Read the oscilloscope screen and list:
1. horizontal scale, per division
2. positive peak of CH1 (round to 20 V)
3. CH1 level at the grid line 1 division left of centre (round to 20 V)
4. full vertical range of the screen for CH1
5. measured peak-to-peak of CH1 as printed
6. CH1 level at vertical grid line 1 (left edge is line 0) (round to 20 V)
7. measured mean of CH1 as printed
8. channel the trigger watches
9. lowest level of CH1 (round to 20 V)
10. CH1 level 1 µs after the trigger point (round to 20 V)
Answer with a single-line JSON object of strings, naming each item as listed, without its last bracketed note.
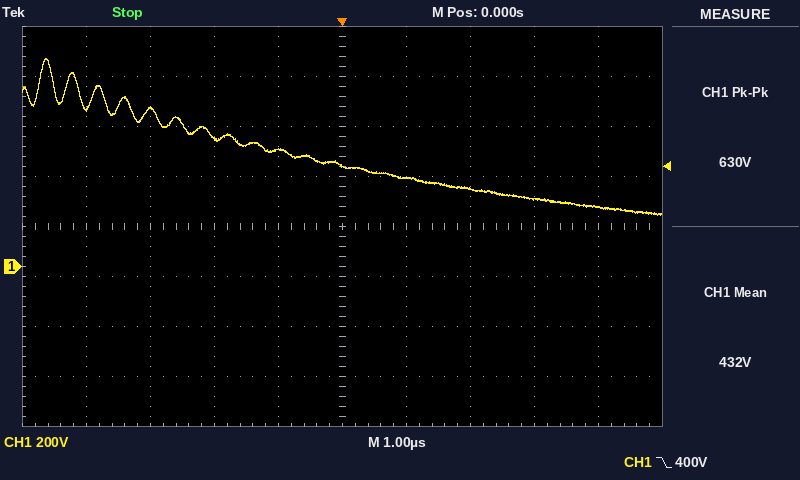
{"horizontal scale, per division": "1 µs", "positive peak of CH1": "840 V", "CH1 level at the grid line 1 division left of centre": "460 V", "full vertical range of the screen for CH1": "1.6 kV", "measured peak-to-peak of CH1 as printed": "630 V", "CH1 level at vertical grid line 1 (left edge is line 0)": "640 V", "measured mean of CH1 as printed": "432 V", "channel the trigger watches": "CH1", "lowest level of CH1": "200 V", "CH1 level 1 µs after the trigger point": "360 V"}
